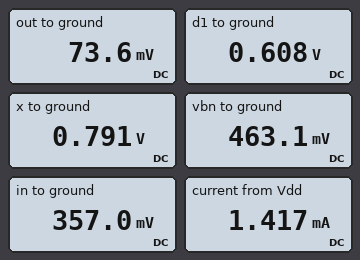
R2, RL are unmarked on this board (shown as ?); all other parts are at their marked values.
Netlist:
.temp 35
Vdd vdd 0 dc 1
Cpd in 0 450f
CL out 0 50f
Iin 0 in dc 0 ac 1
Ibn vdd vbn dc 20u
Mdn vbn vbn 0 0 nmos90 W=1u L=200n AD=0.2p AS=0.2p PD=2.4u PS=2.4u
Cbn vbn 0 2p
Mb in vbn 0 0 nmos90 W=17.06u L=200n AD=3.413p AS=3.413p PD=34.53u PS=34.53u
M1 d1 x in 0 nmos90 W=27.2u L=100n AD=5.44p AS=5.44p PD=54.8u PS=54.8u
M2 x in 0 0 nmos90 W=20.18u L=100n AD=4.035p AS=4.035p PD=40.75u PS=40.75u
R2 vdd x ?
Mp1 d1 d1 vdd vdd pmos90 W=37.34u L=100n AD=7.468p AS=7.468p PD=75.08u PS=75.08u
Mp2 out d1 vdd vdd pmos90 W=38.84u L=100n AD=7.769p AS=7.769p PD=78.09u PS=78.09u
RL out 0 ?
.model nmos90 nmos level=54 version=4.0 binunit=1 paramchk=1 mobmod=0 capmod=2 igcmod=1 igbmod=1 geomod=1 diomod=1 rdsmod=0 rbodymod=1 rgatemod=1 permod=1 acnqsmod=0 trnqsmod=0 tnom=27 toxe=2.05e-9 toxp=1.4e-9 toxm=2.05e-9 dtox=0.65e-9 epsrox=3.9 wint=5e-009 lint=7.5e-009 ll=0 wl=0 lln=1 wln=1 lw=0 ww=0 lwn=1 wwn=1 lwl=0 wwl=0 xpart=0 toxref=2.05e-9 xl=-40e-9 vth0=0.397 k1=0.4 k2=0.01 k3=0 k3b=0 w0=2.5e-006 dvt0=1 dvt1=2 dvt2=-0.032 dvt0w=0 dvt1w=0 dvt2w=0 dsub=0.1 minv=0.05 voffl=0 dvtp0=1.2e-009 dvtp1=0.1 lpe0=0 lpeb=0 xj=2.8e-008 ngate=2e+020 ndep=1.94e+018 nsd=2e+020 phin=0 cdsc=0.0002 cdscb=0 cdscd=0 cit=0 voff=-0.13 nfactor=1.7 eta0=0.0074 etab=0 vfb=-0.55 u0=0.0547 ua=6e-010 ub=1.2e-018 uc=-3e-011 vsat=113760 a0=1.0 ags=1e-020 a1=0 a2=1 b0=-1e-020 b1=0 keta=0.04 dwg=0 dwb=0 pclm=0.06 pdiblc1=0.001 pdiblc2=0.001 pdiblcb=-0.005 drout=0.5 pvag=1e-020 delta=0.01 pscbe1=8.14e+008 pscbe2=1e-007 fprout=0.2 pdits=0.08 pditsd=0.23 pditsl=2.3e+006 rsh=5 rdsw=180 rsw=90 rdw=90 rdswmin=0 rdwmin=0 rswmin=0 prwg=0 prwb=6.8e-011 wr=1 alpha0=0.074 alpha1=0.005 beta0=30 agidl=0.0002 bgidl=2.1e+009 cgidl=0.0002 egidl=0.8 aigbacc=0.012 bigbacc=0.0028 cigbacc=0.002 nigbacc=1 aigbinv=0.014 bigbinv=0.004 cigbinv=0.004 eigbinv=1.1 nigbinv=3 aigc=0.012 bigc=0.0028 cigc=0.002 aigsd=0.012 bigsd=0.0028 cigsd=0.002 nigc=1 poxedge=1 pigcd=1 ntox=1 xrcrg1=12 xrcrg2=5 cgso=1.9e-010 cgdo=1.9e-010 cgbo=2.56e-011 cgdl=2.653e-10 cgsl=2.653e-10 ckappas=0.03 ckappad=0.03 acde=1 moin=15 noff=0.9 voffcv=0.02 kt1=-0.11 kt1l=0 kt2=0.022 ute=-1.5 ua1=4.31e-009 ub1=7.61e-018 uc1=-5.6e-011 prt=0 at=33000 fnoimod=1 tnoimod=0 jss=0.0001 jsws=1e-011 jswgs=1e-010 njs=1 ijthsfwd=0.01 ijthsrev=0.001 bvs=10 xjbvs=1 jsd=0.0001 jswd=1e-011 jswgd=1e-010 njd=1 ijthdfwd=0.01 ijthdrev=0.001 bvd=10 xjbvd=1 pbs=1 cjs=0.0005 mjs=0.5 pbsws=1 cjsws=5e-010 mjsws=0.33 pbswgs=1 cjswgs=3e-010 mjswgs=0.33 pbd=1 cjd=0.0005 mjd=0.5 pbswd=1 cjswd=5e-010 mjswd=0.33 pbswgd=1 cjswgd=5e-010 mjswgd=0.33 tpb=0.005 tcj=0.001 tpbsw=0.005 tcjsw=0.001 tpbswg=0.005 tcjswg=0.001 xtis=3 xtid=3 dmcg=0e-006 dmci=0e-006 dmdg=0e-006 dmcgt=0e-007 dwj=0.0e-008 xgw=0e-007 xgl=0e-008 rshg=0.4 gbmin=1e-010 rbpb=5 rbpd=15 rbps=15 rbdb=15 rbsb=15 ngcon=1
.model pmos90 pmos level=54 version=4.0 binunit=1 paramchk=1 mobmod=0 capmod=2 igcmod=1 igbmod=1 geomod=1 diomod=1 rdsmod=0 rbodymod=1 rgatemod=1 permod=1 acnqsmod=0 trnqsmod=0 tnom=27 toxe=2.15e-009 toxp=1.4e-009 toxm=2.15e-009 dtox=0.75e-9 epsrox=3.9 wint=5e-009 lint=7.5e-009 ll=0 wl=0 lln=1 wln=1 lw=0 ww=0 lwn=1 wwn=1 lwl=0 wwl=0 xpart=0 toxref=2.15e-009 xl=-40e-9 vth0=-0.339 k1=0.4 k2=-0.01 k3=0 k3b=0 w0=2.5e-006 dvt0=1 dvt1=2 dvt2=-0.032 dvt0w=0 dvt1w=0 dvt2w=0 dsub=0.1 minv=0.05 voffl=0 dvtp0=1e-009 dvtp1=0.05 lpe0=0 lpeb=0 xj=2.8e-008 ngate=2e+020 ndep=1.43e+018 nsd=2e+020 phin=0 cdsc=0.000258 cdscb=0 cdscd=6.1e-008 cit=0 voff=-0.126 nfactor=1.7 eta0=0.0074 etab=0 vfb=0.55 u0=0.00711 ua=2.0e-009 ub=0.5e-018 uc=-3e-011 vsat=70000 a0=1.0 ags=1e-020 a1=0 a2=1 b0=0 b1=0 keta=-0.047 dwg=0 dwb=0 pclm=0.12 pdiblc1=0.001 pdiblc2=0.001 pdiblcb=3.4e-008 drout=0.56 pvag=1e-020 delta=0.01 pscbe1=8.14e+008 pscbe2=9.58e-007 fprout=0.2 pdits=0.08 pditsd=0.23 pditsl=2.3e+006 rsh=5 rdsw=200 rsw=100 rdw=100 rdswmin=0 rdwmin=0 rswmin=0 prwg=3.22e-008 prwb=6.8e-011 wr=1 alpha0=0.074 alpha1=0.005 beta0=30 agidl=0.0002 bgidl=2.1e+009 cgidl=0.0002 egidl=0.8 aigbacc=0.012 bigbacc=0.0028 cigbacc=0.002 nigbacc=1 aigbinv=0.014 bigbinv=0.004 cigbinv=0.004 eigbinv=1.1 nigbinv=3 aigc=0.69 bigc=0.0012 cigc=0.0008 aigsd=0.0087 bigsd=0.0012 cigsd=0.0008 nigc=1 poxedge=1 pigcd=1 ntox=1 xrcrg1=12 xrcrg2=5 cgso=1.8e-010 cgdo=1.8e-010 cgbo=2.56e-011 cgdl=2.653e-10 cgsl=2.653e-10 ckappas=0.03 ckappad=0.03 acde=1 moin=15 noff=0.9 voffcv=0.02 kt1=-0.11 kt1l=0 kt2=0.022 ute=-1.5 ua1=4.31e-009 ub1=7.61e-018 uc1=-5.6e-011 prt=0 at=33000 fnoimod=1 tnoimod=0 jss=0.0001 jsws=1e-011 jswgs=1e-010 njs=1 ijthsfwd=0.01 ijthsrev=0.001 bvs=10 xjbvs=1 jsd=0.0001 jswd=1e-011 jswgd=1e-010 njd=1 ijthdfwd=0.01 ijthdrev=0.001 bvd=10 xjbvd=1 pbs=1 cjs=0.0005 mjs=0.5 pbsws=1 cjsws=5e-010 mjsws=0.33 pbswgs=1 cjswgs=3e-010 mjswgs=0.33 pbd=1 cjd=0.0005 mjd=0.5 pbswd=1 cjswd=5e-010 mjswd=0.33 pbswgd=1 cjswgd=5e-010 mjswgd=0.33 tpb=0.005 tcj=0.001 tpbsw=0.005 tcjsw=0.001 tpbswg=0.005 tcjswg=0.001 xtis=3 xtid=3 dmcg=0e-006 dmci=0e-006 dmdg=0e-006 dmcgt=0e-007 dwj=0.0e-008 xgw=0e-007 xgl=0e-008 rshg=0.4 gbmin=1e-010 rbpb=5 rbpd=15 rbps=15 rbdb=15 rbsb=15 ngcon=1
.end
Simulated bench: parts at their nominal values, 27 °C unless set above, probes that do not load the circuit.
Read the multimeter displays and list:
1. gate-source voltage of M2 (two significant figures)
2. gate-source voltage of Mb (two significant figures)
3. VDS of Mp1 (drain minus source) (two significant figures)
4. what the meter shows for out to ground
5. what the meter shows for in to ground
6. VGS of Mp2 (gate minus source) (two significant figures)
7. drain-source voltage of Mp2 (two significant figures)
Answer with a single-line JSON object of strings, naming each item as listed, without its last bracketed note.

{"gate-source voltage of M2": "360 mV", "gate-source voltage of Mb": "460 mV", "VDS of Mp1 (drain minus source)": "-390 mV", "what the meter shows for out to ground": "73.6 mV", "what the meter shows for in to ground": "357.0 mV", "VGS of Mp2 (gate minus source)": "-390 mV", "drain-source voltage of Mp2": "-930 mV"}
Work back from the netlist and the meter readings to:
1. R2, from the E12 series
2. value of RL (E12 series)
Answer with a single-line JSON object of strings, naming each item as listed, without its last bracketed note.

{"R2, from the E12 series": "470 Ω", "value of RL": "120 Ω"}
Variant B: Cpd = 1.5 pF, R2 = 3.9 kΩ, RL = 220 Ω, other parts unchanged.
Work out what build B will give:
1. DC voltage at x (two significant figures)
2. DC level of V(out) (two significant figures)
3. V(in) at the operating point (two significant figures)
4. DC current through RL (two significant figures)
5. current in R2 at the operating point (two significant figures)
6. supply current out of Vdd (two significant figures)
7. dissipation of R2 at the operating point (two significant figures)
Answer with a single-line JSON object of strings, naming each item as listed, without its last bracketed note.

{"DC voltage at x": "680 mV", "DC level of V(out)": "130 mV", "V(in) at the operating point": "270 mV", "DC current through RL": "580 µA", "current in R2 at the operating point": "81 µA", "supply current out of Vdd": "1.0 mA", "dissipation of R2 at the operating point": "26 µW"}
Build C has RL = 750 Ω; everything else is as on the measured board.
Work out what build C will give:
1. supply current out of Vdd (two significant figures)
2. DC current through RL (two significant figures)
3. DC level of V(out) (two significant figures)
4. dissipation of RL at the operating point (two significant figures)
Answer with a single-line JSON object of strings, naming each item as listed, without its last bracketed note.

{"supply current out of Vdd": "1.3 mA", "DC current through RL": "470 µA", "DC level of V(out)": "350 mV", "dissipation of RL at the operating point": "160 µW"}
